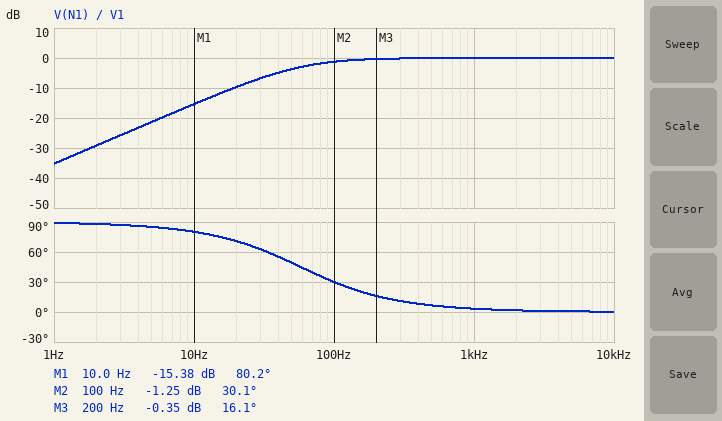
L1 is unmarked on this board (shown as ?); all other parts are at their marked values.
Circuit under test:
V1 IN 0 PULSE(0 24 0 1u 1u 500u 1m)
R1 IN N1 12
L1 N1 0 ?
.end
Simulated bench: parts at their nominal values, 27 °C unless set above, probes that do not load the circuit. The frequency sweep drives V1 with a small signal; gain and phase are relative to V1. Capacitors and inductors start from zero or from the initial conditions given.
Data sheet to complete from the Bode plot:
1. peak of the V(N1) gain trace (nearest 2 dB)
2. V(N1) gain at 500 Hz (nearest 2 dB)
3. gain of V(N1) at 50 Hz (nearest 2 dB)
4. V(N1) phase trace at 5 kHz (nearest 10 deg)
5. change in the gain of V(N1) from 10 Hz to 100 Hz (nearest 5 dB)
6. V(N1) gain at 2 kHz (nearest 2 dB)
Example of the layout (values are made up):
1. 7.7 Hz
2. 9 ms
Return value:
1. 0 dB
2. 0 dB
3. -4 dB
4. 0 deg
5. 15 dB
6. 0 dB
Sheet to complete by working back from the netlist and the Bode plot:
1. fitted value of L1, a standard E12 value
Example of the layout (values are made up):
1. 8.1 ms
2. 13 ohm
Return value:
1. 33 mH
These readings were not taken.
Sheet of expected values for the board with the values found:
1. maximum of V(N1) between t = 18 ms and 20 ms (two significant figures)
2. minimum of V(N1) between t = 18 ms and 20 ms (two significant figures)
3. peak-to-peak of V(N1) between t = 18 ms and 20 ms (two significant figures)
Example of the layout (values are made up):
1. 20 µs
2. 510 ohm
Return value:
1. 13 V
2. -13 V
3. 26 V
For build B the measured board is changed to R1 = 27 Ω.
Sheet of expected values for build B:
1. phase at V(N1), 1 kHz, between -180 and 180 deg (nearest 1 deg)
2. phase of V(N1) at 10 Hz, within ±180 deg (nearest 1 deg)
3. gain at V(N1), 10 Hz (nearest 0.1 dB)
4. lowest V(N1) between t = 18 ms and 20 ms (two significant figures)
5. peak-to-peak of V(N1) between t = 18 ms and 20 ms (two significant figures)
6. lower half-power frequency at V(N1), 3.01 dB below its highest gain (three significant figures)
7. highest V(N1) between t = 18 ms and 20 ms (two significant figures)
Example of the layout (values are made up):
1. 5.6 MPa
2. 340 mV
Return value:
1. 7 deg
2. 86 deg
3. -22.3 dB
4. -14 V
5. 29 V
6. 130 Hz
7. 14 V
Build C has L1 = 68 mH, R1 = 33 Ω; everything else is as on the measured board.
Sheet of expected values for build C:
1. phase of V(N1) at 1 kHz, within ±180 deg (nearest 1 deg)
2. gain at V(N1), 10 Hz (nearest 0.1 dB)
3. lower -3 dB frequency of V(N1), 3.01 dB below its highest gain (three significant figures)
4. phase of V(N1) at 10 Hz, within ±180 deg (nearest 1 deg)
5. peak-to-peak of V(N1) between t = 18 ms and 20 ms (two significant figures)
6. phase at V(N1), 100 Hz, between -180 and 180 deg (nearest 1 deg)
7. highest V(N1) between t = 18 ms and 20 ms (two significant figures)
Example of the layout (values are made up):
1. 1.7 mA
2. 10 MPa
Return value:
1. 4 deg
2. -17.8 dB
3. 77.2 Hz
4. 83 deg
5. 27 V
6. 38 deg
7. 13 V
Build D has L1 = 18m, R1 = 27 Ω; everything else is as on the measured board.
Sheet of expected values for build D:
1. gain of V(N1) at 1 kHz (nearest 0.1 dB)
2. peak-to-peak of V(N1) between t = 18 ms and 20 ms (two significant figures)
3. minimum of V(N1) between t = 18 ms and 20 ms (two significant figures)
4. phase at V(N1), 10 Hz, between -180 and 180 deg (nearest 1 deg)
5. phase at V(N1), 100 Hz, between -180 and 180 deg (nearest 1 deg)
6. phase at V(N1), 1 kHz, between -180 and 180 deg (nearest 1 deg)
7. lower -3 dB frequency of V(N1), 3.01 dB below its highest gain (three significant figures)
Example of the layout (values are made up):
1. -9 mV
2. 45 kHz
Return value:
1. -0.2 dB
2. 33 V
3. -16 V
4. 88 deg
5. 67 deg
6. 13 deg
7. 239 Hz
